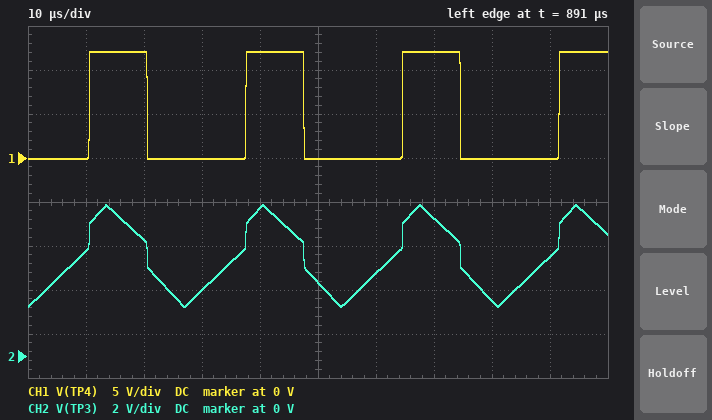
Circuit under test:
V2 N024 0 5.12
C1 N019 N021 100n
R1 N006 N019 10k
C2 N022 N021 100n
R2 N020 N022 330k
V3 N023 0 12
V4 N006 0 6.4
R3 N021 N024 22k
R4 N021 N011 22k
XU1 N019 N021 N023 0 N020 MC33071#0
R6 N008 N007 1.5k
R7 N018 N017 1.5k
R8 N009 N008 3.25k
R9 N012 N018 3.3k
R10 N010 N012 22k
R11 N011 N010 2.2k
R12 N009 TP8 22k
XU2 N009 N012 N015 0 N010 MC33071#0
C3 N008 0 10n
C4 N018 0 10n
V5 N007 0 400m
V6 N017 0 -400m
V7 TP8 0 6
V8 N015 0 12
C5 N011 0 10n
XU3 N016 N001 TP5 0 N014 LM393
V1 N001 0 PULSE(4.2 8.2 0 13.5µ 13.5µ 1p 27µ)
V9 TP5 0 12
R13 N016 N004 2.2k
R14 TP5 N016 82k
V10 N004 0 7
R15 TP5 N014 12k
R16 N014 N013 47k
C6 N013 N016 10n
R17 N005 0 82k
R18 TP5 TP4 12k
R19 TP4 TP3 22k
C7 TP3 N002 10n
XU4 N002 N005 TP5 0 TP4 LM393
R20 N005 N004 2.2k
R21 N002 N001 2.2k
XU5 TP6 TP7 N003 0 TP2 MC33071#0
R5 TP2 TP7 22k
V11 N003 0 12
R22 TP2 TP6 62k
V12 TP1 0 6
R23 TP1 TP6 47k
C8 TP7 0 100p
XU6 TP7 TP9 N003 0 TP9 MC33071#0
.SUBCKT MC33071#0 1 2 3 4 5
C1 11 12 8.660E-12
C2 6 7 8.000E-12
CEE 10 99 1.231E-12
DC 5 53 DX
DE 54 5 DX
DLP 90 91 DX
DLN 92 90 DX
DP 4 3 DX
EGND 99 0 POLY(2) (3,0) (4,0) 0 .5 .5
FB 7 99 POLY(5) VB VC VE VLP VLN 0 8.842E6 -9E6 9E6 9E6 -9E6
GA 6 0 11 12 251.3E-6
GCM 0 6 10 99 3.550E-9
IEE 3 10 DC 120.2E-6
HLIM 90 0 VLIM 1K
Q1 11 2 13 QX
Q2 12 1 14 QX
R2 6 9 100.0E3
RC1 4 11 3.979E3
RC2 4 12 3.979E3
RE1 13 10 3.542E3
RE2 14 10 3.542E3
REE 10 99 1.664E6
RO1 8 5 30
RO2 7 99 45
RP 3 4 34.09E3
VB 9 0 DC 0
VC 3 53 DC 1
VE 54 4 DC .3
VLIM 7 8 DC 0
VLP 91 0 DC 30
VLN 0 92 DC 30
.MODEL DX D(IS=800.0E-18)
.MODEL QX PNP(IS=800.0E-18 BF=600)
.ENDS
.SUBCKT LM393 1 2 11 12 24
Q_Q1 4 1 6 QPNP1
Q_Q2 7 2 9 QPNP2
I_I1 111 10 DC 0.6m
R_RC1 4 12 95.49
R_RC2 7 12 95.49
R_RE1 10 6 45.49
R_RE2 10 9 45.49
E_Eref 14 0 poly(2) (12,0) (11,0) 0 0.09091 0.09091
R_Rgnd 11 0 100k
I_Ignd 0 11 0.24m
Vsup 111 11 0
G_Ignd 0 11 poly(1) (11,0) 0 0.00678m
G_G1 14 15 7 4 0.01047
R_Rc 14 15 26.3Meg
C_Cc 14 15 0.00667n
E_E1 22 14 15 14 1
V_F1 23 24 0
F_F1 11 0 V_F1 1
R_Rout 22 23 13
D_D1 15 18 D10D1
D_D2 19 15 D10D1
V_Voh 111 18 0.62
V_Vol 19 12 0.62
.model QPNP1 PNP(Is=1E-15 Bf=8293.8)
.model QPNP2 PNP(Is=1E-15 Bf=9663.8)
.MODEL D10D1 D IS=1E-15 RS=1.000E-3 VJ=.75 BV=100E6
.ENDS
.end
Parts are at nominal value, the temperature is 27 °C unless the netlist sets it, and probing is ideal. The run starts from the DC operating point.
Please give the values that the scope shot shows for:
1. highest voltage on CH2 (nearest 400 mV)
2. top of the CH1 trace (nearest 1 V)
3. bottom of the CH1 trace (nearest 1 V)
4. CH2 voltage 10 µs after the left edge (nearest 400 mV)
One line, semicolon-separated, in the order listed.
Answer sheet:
6.8 V; 12 V; 0 V; 4.8 V
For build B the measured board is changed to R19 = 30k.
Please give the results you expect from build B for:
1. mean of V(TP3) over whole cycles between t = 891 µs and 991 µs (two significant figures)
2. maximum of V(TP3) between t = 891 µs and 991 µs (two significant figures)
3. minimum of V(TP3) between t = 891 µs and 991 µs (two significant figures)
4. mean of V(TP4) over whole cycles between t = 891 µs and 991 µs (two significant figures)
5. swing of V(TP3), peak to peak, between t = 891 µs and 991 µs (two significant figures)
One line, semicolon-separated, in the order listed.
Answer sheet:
4.3 V; 6.7 V; 2.1 V; 4.4 V; 4.5 V
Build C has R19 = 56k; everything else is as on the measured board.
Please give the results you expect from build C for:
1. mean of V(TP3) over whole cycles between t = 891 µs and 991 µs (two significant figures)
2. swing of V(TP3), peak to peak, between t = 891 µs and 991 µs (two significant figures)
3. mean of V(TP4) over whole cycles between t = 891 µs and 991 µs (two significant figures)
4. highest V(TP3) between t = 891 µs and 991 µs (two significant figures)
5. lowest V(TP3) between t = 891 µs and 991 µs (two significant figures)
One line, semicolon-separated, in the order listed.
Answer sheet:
3.9 V; 4.4 V; 4.3 V; 6.1 V; 1.8 V
